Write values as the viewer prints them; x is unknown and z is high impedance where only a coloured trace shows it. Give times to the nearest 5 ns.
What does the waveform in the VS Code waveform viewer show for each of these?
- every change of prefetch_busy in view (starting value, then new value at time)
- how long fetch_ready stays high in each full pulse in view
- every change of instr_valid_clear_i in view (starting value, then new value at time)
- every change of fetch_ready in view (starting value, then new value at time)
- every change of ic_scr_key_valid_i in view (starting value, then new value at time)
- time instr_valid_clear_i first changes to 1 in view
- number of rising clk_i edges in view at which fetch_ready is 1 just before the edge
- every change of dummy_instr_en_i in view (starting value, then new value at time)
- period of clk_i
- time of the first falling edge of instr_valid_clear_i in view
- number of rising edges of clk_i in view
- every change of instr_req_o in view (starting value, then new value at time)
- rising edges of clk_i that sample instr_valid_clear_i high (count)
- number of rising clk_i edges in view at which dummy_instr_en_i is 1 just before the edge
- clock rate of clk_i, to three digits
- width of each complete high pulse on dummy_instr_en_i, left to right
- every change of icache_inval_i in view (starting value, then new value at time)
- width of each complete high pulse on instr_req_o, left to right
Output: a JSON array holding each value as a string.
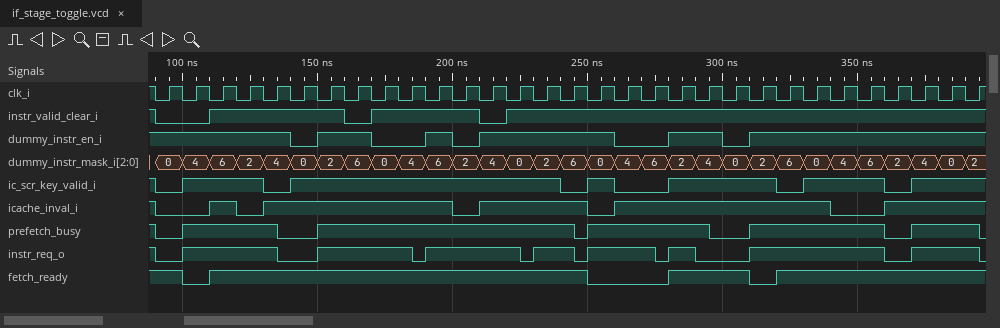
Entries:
["1, 0 at 90 ns, 1 at 100 ns, 0 at 135 ns, 1 at 150 ns, 0 at 245 ns, 1 at 250 ns, 0 at 295 ns, 1 at 310 ns, 0 at 360 ns, 1 at 370 ns, 0 at 395 ns", "140 ns, 30 ns", "1, 0 at 90 ns, 1 at 110 ns, 0 at 160 ns, 1 at 170 ns, 0 at 210 ns, 1 at 220 ns", "1, 0 at 100 ns, 1 at 110 ns, 0 at 250 ns, 1 at 280 ns, 0 at 310 ns, 1 at 320 ns", "1, 0 at 90 ns, 1 at 100 ns, 0 at 130 ns, 1 at 140 ns, 0 at 240 ns, 1 at 250 ns, 0 at 260 ns, 1 at 280 ns, 0 at 320 ns, 1 at 330 ns, 0 at 360 ns, 1 at 370 ns", "110 ns", "26", "1, 0 at 140 ns, 1 at 150 ns, 0 at 170 ns, 1 at 190 ns, 0 at 200 ns, 1 at 210 ns, 0 at 260 ns, 1 at 280 ns, 0 at 300 ns, 1 at 310 ns", "10 ns", "90 ns", "31", "1, 0 at 90 ns, 1 at 100 ns, 0 at 135 ns, 1 at 150 ns, 0 at 185 ns, 1 at 190 ns, 0 at 225 ns, 1 at 230 ns, 0 at 245 ns, 1 at 250 ns, 0 at 275 ns, 1 at 280 ns, 0 at 290 ns, 1 at 310 ns, 0 at 360 ns, 1 at 370 ns, 0 at 395 ns", "27", "24", "100 MHz", "20 ns, 10 ns, 50 ns, 20 ns", "1, 0 at 90 ns, 1 at 110 ns, 0 at 120 ns, 1 at 130 ns, 0 at 200 ns, 1 at 210 ns, 0 at 250 ns, 1 at 260 ns, 0 at 340 ns, 1 at 360 ns", "35 ns, 35 ns, 35 ns, 15 ns, 25 ns, 10 ns, 50 ns, 25 ns"]
